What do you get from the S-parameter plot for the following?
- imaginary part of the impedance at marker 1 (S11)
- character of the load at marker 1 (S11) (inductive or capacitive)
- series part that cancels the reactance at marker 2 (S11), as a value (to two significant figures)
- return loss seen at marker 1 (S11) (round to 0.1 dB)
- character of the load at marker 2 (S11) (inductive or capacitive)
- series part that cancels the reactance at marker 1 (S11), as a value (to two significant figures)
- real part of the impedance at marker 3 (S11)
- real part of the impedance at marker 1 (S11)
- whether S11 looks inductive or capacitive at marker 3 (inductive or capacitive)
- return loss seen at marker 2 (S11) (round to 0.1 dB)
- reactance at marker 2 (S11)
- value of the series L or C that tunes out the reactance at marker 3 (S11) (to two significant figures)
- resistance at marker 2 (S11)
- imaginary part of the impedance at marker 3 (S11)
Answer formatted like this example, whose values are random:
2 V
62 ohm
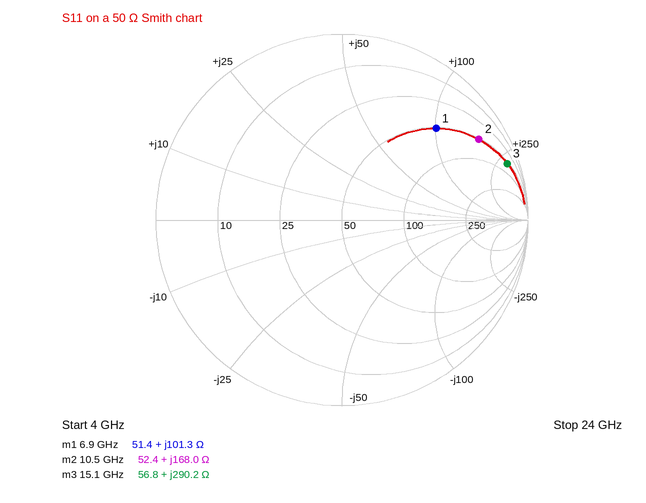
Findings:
+101.3 Ω
inductive
90 fF
3.0 dB
inductive
230 fF
56.8 Ω
51.4 Ω
inductive
1.4 dB
+168.0 Ω
36 fF
52.4 Ω
+290.2 Ω
